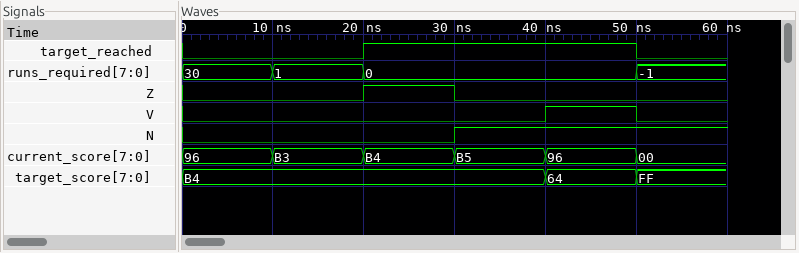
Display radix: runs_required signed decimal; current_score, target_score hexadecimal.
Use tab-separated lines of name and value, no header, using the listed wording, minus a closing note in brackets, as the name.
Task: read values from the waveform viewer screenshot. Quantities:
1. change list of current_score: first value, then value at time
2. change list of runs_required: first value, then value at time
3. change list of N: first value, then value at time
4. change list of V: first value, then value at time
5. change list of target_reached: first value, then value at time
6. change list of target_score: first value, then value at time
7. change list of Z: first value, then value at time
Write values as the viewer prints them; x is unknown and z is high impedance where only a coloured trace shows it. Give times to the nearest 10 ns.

change list of current_score: first value, then value at time	96, B3 at 10 ns, B4 at 20 ns, B5 at 30 ns, 96 at 40 ns, 00 at 50 ns
change list of runs_required: first value, then value at time	30, 1 at 10 ns, 0 at 20 ns, -1 at 50 ns
change list of N: first value, then value at time	0, 1 at 30 ns
change list of V: first value, then value at time	0, 1 at 40 ns, 0 at 50 ns
change list of target_reached: first value, then value at time	0, 1 at 20 ns, 0 at 50 ns
change list of target_score: first value, then value at time	B4, 64 at 40 ns, FF at 50 ns
change list of Z: first value, then value at time	0, 1 at 20 ns, 0 at 30 ns
